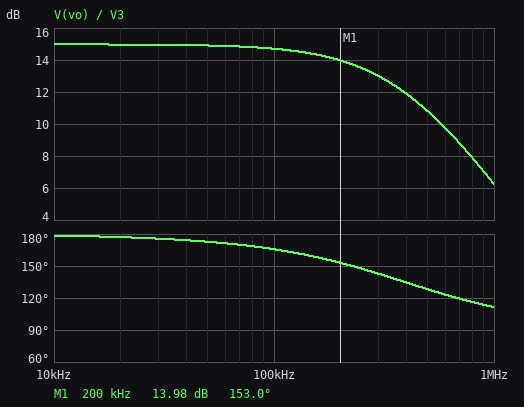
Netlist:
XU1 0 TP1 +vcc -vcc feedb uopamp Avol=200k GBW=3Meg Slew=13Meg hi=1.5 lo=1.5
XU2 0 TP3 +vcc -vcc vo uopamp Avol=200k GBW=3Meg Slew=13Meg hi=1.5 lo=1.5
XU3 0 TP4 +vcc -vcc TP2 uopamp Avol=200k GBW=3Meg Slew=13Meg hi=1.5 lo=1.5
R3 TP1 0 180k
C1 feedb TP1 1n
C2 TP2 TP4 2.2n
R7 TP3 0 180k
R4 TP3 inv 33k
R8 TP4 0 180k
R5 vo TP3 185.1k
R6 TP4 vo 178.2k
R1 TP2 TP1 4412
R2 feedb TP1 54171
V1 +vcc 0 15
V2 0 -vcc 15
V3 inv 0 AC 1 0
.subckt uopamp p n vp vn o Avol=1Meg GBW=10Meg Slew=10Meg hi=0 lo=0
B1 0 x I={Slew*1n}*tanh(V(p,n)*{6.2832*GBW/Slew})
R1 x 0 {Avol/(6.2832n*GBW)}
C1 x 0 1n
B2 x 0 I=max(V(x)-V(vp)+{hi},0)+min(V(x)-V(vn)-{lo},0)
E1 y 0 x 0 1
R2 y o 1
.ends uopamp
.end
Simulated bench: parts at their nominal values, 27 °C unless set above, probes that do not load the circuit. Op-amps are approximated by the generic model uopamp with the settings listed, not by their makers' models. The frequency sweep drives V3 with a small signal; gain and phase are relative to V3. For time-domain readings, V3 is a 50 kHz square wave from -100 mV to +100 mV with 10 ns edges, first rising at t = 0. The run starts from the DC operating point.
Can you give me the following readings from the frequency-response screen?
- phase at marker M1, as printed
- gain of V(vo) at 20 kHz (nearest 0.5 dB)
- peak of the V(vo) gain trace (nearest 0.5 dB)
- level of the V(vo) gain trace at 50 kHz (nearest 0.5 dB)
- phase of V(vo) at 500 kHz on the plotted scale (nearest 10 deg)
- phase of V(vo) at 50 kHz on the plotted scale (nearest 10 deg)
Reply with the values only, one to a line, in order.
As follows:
153.0 deg
15.0 dB
15.0 dB
15.0 dB
130 deg
170 deg
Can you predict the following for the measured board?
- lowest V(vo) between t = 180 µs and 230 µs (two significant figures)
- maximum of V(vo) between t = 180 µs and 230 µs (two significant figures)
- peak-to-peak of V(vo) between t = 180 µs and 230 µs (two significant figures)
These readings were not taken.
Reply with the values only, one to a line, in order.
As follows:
-560 mV
560 mV
1.1 V
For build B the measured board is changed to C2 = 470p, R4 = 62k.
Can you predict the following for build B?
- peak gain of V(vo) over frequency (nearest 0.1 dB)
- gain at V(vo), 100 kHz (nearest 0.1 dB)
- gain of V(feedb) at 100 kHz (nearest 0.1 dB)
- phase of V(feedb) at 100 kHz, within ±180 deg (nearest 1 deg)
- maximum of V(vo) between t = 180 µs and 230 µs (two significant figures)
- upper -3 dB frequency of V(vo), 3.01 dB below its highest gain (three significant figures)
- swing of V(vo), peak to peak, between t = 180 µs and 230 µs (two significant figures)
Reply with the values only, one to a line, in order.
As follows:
9.5 dB
9.4 dB
-34.0 dB
-12 deg
300 mV
598 kHz
600 mV
